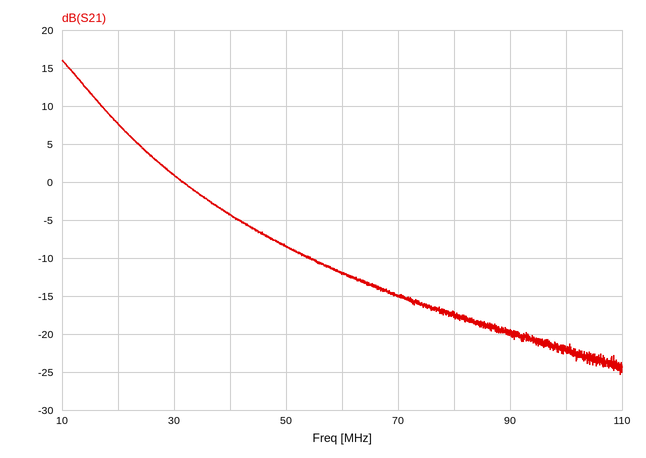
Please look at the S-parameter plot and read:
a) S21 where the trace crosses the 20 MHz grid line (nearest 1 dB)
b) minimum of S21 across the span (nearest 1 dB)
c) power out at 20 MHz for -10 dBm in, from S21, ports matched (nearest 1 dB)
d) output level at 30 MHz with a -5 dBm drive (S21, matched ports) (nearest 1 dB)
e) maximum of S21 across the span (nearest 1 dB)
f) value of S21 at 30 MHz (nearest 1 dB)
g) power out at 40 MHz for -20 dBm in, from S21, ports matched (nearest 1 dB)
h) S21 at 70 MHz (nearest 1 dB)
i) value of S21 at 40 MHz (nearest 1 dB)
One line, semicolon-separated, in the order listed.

8 dB; -25 dB; -2 dBm; -4 dBm; 16 dB; 1 dB; -24 dBm; -15 dB; -4 dB
